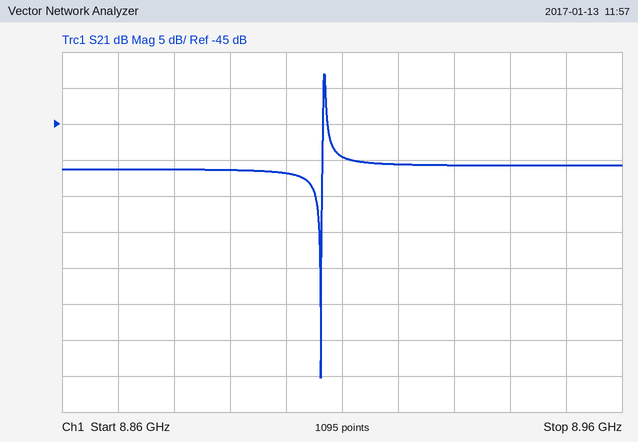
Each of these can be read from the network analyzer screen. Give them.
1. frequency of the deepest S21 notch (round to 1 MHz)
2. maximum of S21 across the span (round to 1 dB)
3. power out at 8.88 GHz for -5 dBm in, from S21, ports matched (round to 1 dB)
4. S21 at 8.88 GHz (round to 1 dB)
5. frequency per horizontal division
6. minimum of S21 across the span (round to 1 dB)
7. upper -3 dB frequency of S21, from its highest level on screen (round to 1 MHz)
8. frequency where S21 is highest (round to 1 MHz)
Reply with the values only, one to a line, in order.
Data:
8.906 GHz
-38 dB
-56 dBm
-51 dB
10 MHz
-80 dB
8.907 GHz
8.907 GHz
